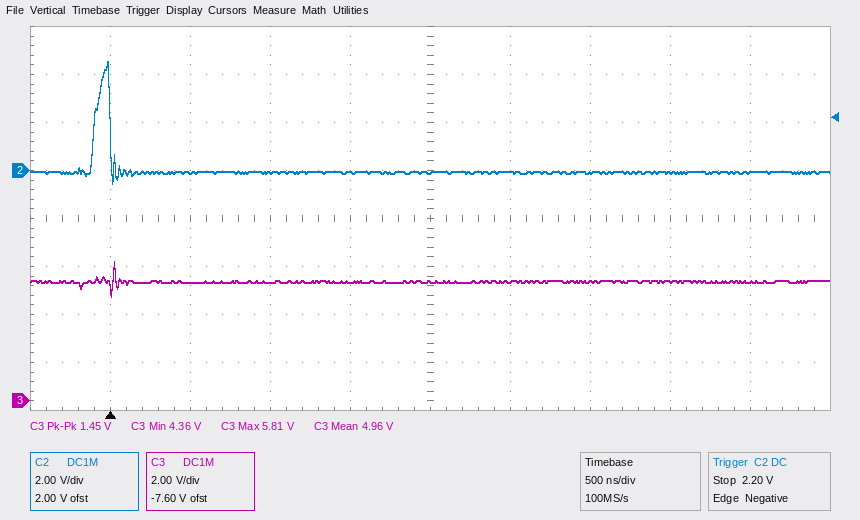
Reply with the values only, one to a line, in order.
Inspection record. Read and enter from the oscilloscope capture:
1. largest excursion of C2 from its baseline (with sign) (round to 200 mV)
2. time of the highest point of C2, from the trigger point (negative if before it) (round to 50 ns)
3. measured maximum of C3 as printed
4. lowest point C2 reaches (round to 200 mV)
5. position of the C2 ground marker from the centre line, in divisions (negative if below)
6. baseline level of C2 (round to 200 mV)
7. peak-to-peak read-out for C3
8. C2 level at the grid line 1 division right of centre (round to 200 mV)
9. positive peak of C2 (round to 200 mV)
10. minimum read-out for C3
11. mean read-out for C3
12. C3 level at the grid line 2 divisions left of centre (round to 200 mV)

+4.6 V
0 ns
5.81 V
-600 mV
+1.0 div
0.0 V
1.45 V
0.0 V
4.6 V
4.36 V
4.96 V
5.0 V
